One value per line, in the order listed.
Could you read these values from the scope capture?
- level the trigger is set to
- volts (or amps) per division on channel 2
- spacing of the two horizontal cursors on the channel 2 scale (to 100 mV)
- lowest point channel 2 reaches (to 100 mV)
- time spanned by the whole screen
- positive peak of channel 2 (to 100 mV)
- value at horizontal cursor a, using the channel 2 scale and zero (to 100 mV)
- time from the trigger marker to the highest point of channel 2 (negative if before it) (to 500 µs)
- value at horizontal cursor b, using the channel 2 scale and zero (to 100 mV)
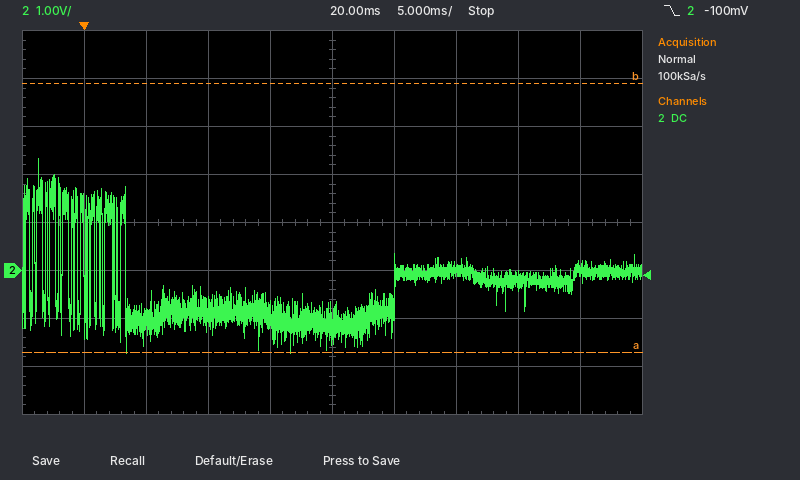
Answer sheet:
-100 mV
1 V
5.6 V
-1.7 V
50 ms
2.3 V
-1.7 V
-3.5 ms
3.9 V
